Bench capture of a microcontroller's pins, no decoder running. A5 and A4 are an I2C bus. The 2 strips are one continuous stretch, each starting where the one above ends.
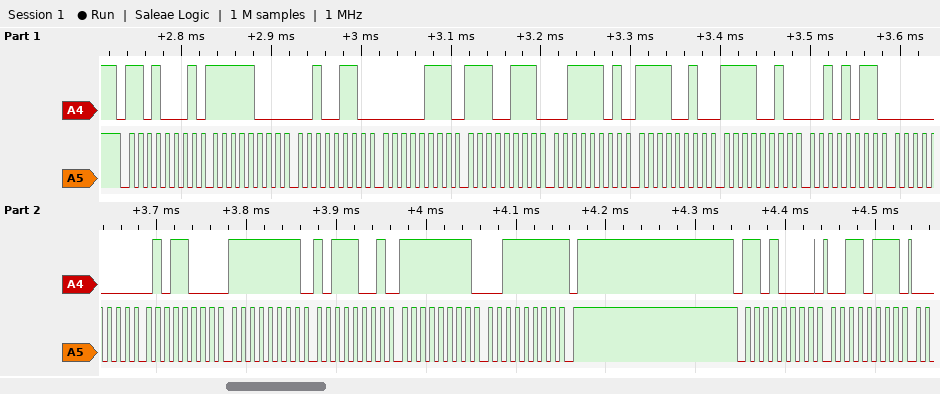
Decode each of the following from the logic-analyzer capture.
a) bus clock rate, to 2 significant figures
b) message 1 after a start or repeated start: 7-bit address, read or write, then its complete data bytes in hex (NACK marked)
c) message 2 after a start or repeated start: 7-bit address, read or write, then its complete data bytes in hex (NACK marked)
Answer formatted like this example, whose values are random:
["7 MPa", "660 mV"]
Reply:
["100 kHz", "0x68 read: F8 26 07 E7 3D F2 F2 2B 00 58 FF B9 FF 3F NACK", "0x68 write: 37"]
